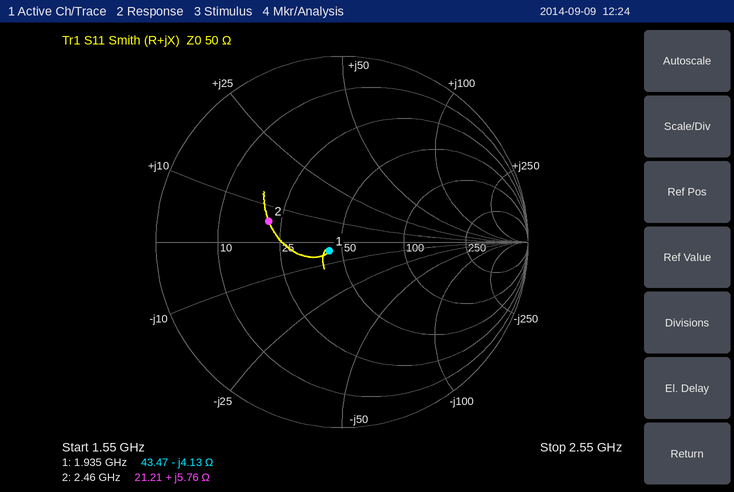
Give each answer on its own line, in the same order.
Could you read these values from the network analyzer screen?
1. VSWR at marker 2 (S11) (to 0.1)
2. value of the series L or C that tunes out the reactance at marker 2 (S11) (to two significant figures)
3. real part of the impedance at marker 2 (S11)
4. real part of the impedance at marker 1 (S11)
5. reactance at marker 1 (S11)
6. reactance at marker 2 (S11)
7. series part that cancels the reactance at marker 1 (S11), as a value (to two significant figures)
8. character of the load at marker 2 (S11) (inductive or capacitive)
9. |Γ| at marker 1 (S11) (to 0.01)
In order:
2.4
11 pF
21.21 Ω
43.47 Ω
-4.13 Ω
+5.76 Ω
340 pH
inductive
0.08
